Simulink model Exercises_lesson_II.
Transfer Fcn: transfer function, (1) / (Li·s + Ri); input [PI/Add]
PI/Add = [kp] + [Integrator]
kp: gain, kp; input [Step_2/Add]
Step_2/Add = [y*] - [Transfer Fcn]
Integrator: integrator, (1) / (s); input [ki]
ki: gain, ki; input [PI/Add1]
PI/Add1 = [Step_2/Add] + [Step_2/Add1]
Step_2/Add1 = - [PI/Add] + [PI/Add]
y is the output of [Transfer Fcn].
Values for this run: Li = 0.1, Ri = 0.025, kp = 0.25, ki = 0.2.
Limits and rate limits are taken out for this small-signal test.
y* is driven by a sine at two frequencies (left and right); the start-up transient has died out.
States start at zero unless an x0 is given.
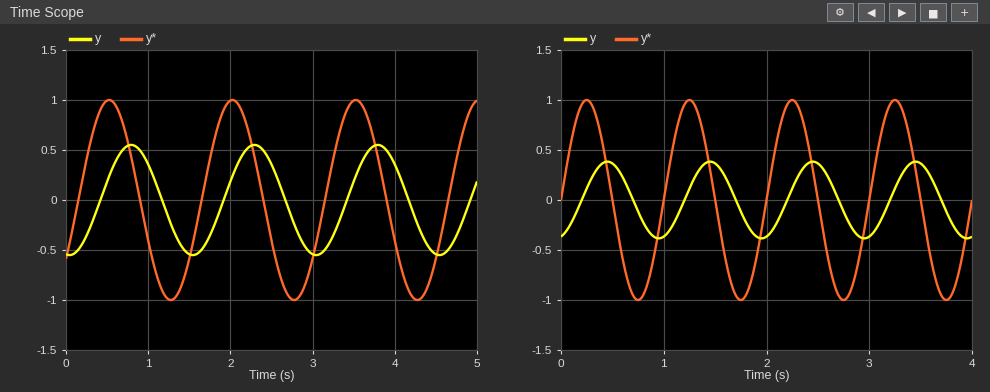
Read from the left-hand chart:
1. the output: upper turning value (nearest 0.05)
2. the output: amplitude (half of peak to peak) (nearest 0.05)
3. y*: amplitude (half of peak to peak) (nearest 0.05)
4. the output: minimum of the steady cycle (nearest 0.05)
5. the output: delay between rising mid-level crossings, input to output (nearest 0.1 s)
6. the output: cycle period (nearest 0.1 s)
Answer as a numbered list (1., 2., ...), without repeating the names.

1. 0.55
2. 0.55
3. 1.00
4. -0.55
5. 0.3 s
6. 1.5 s
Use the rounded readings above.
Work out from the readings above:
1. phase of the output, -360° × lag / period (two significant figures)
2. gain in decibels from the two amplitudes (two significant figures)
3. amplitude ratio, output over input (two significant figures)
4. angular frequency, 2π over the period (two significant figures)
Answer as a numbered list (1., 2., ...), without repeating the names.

1. -72°
2. -5.2 dB
3. 0.55
4. 4.2 rad/s
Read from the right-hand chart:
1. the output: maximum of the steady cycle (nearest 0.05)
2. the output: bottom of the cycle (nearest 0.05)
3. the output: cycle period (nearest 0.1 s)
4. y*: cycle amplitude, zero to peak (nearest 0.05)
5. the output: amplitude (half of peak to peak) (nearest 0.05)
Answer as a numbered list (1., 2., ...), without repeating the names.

1. 0.40
2. -0.40
3. 1.0 s
4. 1.00
5. 0.40
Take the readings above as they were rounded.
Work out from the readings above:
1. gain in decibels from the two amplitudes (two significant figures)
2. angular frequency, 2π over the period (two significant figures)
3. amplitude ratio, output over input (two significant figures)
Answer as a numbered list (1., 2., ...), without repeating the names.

1. -8.0 dB
2. 6.3 rad/s
3. 0.40
